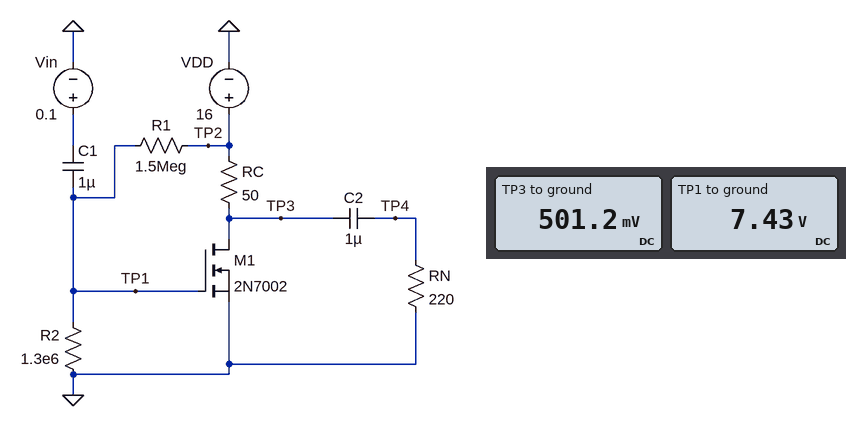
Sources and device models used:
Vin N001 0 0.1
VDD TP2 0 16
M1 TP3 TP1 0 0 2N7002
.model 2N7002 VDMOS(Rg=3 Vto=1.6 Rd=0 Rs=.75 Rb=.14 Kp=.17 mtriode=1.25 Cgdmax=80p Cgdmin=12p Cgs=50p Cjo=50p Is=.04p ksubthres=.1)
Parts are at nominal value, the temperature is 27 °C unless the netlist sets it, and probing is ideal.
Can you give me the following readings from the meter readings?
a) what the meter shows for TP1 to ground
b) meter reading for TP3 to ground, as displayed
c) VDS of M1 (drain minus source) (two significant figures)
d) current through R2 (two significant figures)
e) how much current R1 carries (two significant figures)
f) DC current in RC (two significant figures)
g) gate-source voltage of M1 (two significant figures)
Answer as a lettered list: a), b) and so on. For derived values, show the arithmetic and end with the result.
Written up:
a) 7.43 V
b) 501.2 mV
c) 501.2 mV = 500 mV
d) (7.43 V) / 1.3 MΩ = 5.7 µA
e) (16 V - 7.43 V) / 1.5 MΩ = 5.7 µA
f) (16 V - 501.2 mV) / 50 Ω = 310 mA
g) 7.43 V = 7.4 V
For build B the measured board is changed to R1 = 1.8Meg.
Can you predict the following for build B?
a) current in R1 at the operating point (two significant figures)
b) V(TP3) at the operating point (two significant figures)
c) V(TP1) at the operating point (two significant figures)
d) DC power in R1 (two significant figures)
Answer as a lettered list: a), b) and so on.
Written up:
a) 5.2 µA
b) 540 mV
c) 6.7 V
d) 48 µW
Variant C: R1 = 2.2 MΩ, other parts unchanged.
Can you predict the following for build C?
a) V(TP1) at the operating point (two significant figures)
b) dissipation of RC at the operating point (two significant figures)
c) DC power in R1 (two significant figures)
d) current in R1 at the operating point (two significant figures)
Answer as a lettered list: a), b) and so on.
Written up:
a) 5.9 V
b) 4.7 W
c) 46 µW
d) 4.6 µA
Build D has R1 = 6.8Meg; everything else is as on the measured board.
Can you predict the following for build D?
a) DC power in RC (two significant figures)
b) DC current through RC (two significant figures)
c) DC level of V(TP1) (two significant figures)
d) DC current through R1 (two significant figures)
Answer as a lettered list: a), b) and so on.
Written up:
a) 250 mW
b) 71 mA
c) 2.6 V
d) 2.0 µA
